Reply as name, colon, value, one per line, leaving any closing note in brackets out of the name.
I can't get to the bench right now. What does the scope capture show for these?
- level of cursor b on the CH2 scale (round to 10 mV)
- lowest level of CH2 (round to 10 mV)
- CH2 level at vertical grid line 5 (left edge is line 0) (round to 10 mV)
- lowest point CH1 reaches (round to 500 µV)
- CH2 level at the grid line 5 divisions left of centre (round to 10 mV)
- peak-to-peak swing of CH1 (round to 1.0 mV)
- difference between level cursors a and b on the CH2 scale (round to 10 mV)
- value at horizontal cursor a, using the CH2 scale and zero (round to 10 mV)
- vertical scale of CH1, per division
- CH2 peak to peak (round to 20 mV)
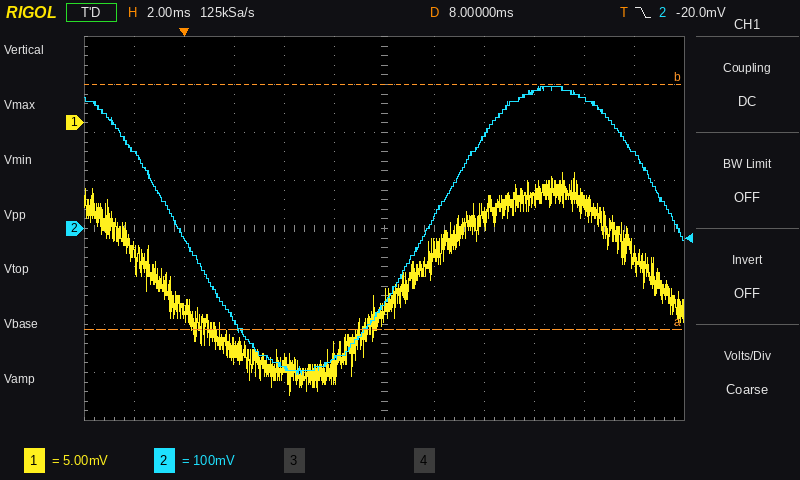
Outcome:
level of cursor b on the CH2 scale: 300 mV
lowest level of CH2: -300 mV
CH2 level at vertical grid line 5 (left edge is line 0): -270 mV
lowest point CH1 reaches: -28.5 mV
CH2 level at the grid line 5 divisions left of centre: 160 mV
peak-to-peak swing of CH1: 23.0 mV
difference between level cursors a and b on the CH2 scale: 510 mV
value at horizontal cursor a, using the CH2 scale and zero: -210 mV
vertical scale of CH1, per division: 5 mV
CH2 peak to peak: 600 mV
